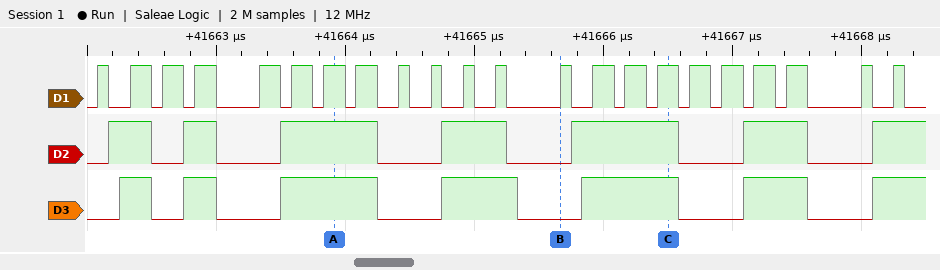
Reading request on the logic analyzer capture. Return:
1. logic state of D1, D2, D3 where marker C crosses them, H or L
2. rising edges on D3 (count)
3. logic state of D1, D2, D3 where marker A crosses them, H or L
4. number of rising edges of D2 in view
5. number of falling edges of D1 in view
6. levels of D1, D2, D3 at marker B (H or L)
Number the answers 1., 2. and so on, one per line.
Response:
1. D1=H, D2=H, D3=H
2. 7
3. D1=H, D2=H, D3=H
4. 7
5. 22
6. D1=H, D2=L, D3=L
